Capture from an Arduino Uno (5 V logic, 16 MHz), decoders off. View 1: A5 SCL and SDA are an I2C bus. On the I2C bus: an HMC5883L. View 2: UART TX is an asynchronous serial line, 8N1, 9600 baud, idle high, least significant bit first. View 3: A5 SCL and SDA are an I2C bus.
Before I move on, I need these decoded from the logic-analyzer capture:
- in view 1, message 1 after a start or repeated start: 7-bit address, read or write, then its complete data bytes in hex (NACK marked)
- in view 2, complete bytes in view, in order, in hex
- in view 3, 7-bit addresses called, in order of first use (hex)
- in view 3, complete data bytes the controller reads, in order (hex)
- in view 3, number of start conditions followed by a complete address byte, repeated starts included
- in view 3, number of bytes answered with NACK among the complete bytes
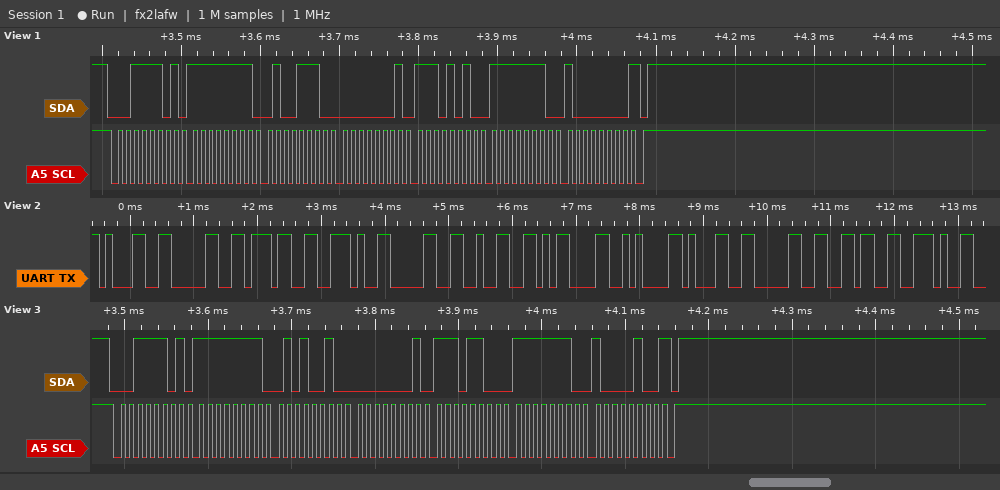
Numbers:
0x1E read: FF 4E 01 EA FE 80 NACK
31 30 37 2E 30 32 0D 0A 31 30 36 2E
0x1E
FF 52 01 EC FE 84
1
1
